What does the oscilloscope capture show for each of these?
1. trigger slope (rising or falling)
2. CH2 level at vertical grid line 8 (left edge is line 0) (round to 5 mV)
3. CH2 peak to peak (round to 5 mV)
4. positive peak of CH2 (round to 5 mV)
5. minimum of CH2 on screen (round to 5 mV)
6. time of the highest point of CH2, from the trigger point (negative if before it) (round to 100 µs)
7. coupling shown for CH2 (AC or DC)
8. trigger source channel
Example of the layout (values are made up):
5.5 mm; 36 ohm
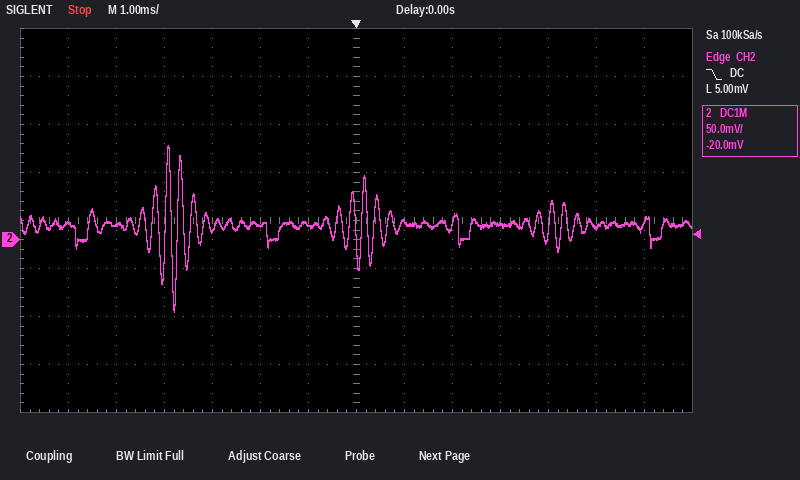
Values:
falling; 20 mV; 175 mV; 100 mV; -75 mV; -3.9 ms; DC; CH2
